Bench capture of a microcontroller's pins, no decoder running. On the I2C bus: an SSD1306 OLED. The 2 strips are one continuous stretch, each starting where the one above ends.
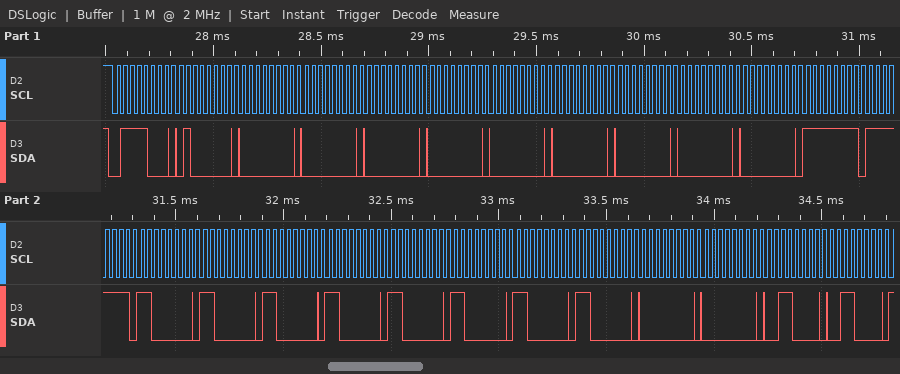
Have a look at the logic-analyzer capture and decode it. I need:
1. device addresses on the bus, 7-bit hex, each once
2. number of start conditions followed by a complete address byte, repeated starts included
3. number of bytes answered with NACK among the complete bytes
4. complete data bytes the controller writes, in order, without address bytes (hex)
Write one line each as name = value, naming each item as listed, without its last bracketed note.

device addresses on the bus, 7-bit hex, each once = 0x3C
number of start conditions followed by a complete address byte, repeated starts included = 1
number of bytes answered with NACK among the complete bytes = 0
complete data bytes the controller writes, in order, without address bytes = 40 00 00 00 00 00 00 00 00 00 FF FF C0 C0 C0 C0 C0 C0 C0 C0 00 00 30 30
